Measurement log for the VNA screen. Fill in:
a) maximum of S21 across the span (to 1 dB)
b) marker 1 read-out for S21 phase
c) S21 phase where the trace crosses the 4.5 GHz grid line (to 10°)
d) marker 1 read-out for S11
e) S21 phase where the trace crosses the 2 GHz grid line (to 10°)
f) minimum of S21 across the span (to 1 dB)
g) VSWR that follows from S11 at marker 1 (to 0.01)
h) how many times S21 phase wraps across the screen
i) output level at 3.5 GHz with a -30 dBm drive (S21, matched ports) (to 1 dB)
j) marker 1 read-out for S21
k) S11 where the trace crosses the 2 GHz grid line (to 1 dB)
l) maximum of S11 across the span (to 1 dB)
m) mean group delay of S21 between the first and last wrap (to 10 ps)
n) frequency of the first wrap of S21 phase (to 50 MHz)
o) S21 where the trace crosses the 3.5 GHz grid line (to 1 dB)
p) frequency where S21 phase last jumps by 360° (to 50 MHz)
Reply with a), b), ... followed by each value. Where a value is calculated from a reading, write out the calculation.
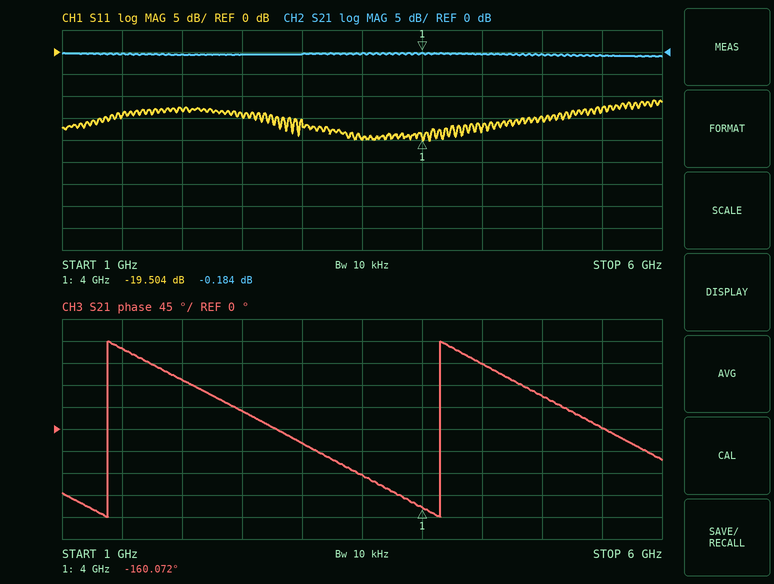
a) 0 dB
b) -160.072°
c) 130°
d) -19.504 dB
e) 100°
f) -1 dB
g) (1 + 0.1059)/(1 − 0.1059) ≈ 1.24
h) 2
i) -30 dBm + (0 dB) = -30 dBm
j) -0.184 dB
k) -13 dB
l) -11 dB
m) 1 cycle / (4.15 GHz − 1.40 GHz) ≈ 364 ps, so 360 ps to the nearest 10 ps
n) 1.40 GHz
o) 0 dB
p) 4.15 GHz
